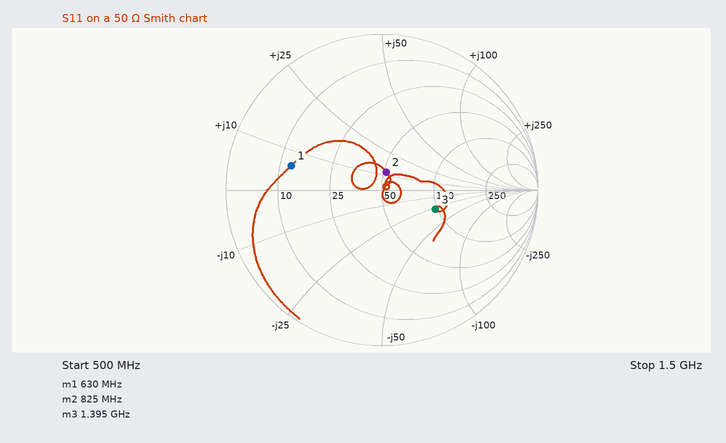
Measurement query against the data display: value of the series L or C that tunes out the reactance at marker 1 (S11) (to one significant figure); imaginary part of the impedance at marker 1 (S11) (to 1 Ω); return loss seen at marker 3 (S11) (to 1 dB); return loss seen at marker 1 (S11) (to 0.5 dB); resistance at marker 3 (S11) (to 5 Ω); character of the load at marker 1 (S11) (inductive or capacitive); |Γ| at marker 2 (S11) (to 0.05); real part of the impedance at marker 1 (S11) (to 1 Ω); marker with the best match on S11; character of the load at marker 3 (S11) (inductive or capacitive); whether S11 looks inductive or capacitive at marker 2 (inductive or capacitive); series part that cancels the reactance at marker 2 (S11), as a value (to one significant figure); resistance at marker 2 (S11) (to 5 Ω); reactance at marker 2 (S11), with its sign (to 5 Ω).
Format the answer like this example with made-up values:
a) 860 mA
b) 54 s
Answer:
a) 40 pF
b) +6 Ω
c) 9 dB
d) 4.5 dB
e) 95 Ω
f) inductive
g) 0.10
h) 13 Ω
i) marker 2
j) capacitive
k) inductive
l) 20 pF
m) 50 Ω
n) +10 Ω
